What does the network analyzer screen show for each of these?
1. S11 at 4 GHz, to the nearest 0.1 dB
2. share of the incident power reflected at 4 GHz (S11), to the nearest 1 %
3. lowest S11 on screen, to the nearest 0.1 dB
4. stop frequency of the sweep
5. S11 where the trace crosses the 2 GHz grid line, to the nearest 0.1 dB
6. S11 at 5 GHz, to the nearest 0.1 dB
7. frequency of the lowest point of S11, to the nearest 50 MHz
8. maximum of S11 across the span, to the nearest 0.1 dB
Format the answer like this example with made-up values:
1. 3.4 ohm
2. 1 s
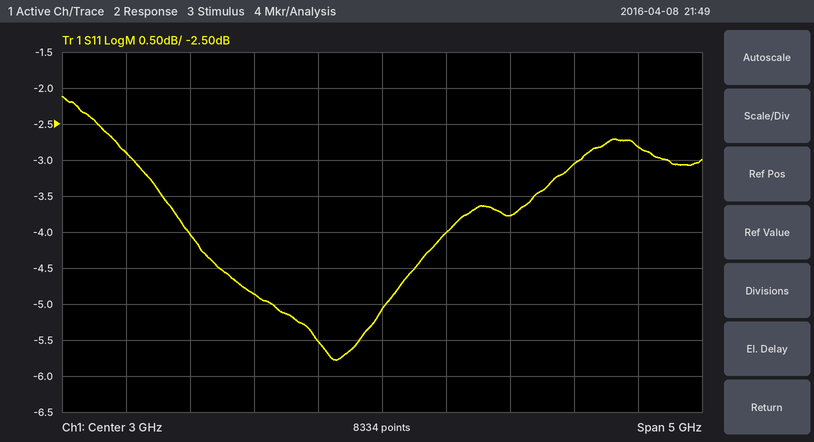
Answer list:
1. -3.8 dB
2. 42 %
3. -5.8 dB
4. 5.5 GHz
5. -4.9 dB
6. -2.8 dB
7. 2.65 GHz
8. -2.1 dB
